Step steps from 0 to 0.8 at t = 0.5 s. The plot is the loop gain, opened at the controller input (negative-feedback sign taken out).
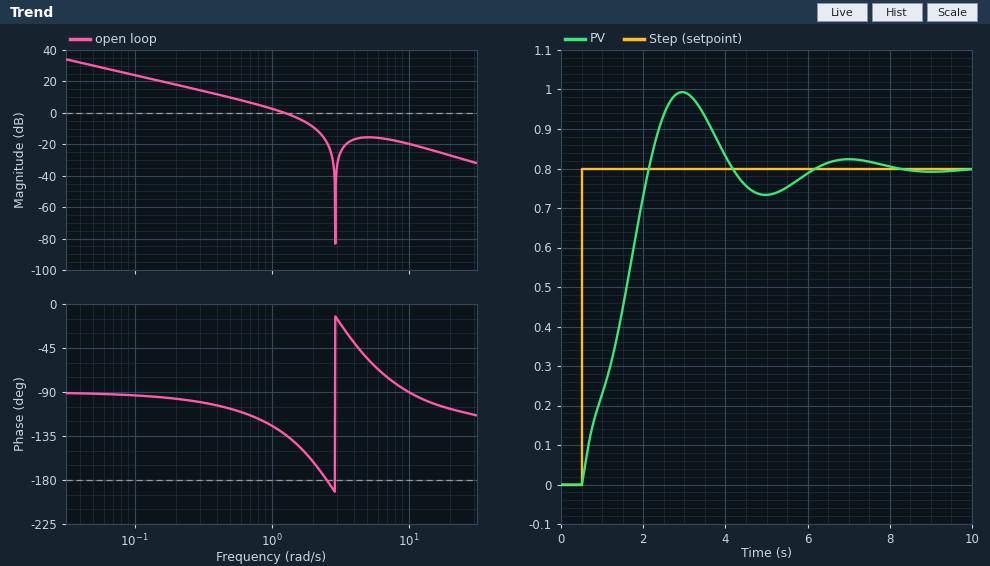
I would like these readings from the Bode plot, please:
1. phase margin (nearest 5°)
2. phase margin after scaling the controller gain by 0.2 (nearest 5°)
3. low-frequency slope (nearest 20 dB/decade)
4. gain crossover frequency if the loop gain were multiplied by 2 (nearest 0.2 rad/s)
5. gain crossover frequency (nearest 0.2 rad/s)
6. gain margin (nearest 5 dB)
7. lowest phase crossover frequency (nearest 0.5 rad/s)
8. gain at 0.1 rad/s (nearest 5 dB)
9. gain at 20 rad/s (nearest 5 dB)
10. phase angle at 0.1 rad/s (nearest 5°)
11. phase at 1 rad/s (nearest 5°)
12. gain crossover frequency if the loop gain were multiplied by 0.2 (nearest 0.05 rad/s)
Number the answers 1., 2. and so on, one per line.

1. 45°
2. 80°
3. -20 dB/decade
4. 1.8 rad/s
5. 1.2 rad/s
6. 20 dB
7. 2.5 rad/s
8. 25 dB
9. -25 dB
10. -95°
11. -125°
12. 0.30 rad/s
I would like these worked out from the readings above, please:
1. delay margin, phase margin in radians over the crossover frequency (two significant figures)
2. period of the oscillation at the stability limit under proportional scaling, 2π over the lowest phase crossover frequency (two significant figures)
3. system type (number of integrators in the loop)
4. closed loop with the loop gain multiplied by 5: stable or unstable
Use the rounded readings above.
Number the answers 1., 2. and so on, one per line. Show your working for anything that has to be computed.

1. 45 × π / 180 / 1.2 = 0.65 s
2. 2π / 2.5 = 2.5 s
3. 1
4. stable
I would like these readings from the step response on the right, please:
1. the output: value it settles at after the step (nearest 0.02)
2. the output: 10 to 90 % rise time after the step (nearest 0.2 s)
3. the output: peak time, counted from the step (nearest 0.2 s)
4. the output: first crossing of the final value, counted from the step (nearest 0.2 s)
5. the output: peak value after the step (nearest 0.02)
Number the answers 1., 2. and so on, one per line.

1. 0.80
2. 1.4 s
3. 2.4 s
4. 1.6 s
5. 1.00
